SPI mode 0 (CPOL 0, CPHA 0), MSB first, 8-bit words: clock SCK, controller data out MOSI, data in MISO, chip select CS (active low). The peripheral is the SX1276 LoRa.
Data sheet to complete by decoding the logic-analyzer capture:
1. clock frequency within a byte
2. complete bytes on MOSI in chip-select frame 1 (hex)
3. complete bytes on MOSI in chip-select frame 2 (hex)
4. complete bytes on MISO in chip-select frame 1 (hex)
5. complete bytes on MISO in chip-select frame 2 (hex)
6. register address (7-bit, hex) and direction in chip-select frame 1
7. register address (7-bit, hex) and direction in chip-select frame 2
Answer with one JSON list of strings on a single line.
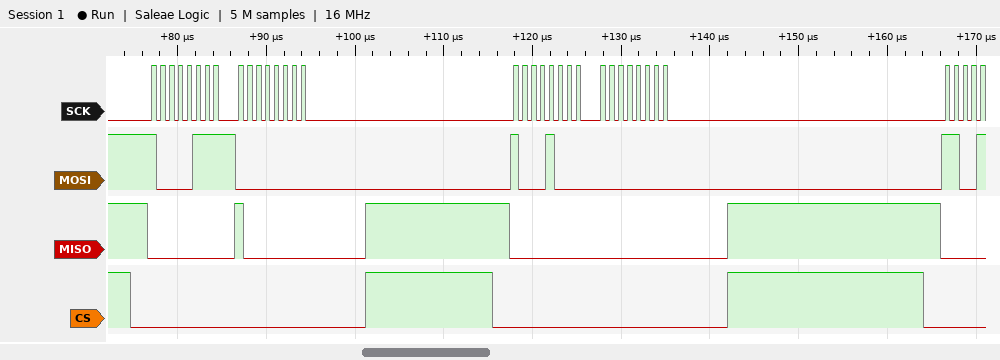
["1 MHz", "87 00", "88 00", "00 80", "00 00", "0x07 write", "0x08 write"]
